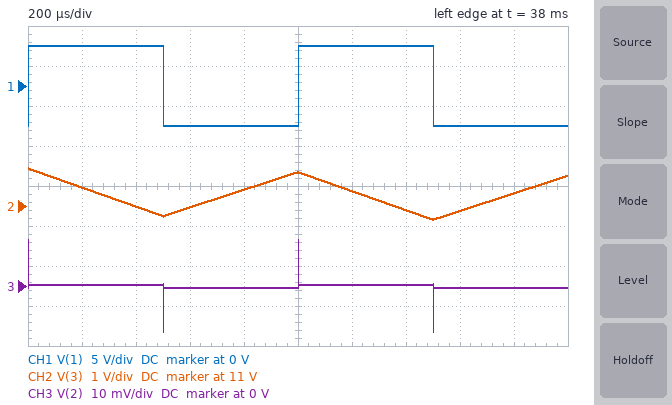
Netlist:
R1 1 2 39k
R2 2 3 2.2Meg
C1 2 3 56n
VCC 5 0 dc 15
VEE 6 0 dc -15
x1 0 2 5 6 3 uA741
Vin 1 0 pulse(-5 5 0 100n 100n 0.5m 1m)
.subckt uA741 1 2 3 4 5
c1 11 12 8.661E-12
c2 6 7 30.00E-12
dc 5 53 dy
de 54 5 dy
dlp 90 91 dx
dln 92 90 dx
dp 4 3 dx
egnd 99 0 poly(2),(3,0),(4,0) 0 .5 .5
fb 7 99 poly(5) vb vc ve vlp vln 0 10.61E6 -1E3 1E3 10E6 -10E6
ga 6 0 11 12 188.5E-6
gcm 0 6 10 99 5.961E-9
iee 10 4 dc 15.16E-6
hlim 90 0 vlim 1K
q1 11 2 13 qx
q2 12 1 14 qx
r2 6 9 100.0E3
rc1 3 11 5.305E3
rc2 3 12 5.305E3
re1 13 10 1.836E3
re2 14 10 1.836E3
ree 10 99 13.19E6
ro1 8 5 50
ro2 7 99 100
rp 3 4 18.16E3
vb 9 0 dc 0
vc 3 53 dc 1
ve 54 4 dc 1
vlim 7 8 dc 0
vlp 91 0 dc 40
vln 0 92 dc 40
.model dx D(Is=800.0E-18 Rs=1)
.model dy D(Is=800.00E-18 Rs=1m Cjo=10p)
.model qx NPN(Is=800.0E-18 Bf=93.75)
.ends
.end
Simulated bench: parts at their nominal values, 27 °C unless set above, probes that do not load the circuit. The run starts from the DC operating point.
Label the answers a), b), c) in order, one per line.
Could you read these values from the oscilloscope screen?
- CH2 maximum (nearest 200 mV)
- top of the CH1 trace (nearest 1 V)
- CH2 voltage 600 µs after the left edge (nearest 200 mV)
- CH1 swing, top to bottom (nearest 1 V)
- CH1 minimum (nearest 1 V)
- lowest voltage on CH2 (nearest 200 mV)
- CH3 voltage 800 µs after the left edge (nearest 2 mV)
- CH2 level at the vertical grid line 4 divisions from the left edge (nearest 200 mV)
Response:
a) 12.0 V
b) 5 V
c) 11.0 V
d) 10 V
e) -5 V
f) 10.6 V
g) 0 V
h) 11.4 V
